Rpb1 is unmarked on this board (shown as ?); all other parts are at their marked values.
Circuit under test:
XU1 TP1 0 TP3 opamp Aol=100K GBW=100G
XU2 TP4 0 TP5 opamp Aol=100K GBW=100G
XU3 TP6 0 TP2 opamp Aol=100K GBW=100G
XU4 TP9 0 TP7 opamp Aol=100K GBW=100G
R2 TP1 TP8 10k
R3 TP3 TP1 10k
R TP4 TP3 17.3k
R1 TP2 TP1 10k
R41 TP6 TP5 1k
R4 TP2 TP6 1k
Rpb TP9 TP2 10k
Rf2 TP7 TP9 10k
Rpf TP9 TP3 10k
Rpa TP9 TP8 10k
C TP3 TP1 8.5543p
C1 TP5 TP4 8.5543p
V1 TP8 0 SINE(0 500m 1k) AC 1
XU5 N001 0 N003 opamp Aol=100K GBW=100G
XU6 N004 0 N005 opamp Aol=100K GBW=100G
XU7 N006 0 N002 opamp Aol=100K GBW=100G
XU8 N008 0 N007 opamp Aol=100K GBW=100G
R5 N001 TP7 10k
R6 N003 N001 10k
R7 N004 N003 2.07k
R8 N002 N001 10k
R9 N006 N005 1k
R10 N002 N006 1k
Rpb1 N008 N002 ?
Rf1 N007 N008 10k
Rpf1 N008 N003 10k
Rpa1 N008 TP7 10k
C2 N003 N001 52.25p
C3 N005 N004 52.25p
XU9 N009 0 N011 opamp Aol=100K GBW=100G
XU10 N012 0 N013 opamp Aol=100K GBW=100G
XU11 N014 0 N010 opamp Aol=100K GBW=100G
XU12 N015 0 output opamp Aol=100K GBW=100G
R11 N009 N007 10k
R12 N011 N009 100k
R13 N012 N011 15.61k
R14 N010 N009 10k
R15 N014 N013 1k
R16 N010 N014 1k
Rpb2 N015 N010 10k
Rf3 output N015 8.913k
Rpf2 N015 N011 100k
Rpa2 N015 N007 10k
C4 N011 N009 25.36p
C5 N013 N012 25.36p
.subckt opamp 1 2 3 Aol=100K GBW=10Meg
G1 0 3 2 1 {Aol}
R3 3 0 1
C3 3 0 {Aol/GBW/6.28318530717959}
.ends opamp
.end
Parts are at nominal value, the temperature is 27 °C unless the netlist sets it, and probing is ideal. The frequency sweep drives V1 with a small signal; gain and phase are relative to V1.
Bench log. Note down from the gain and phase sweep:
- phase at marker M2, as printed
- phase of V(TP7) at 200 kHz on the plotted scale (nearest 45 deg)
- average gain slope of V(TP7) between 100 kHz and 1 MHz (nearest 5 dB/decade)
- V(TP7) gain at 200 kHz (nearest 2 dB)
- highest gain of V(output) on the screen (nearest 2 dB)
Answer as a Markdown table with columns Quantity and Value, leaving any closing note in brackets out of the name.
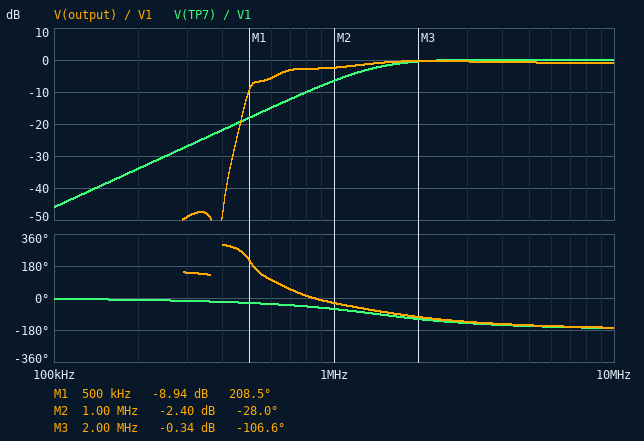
| Quantity | Value |
|---|---|
| phase at marker M2, as printed | -28.0 deg |
| phase of V(TP7) at 200 kHz on the plotted scale | 0 deg |
| average gain slope of V(TP7) between 100 kHz and 1 MHz | 40 dB/decade |
| V(TP7) gain at 200 kHz | -34 dB |
| highest gain of V(output) on the screen | 0 dB |
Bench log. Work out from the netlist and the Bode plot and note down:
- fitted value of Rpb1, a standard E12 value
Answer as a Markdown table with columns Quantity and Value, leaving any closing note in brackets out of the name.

| Quantity | Value |
|---|---|
| fitted value of Rpb1, a standard E12 value | 15 kΩ |
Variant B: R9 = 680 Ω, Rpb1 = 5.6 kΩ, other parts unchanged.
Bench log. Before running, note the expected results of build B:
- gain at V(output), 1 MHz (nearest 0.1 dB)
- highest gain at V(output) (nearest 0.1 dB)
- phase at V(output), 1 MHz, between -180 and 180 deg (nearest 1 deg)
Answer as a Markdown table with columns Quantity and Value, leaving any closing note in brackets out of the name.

| Quantity | Value |
|---|---|
| gain at V(output), 1 MHz | 5.4 dB |
| highest gain at V(output) | 7.1 dB |
| phase at V(output), 1 MHz, between -180 and 180 deg | -15 deg |
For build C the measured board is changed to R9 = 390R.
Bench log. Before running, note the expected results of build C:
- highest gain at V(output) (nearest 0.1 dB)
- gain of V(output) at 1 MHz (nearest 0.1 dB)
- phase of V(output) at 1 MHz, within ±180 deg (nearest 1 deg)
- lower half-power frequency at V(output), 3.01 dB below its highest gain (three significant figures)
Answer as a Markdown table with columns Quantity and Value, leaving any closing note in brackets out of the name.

| Quantity | Value |
|---|---|
| highest gain at V(output) | 3.8 dB |
| gain of V(output) at 1 MHz | 0.2 dB |
| phase of V(output) at 1 MHz, within ±180 deg | 59 deg |
| lower half-power frequency at V(output), 3.01 dB below its highest gain | 1.01 MHz |
